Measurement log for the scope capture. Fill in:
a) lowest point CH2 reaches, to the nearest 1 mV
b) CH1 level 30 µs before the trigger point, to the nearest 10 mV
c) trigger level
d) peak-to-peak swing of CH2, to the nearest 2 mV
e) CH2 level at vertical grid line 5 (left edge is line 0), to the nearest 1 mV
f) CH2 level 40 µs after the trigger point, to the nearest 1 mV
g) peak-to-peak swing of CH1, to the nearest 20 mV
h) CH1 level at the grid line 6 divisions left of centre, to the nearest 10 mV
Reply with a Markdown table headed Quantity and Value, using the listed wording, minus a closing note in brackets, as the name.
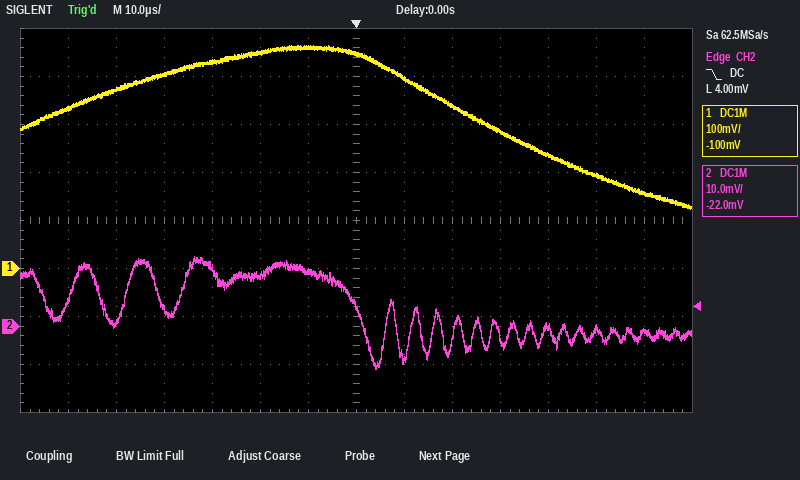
| Quantity | Value |
|---|---|
| lowest point CH2 reaches, to the nearest 1 mV | -9 mV |
| CH1 level 30 µs before the trigger point, to the nearest 10 mV | 430 mV |
| trigger level | 4.00 mV |
| peak-to-peak swing of CH2, to the nearest 2 mV | 24 mV |
| CH2 level at vertical grid line 5 (left edge is line 0), to the nearest 1 mV | 11 mV |
| CH2 level 40 µs after the trigger point, to the nearest 1 mV | 0 mV |
| peak-to-peak swing of CH1, to the nearest 20 mV | 340 mV |
| CH1 level at the grid line 6 divisions left of centre, to the nearest 10 mV | 330 mV |
